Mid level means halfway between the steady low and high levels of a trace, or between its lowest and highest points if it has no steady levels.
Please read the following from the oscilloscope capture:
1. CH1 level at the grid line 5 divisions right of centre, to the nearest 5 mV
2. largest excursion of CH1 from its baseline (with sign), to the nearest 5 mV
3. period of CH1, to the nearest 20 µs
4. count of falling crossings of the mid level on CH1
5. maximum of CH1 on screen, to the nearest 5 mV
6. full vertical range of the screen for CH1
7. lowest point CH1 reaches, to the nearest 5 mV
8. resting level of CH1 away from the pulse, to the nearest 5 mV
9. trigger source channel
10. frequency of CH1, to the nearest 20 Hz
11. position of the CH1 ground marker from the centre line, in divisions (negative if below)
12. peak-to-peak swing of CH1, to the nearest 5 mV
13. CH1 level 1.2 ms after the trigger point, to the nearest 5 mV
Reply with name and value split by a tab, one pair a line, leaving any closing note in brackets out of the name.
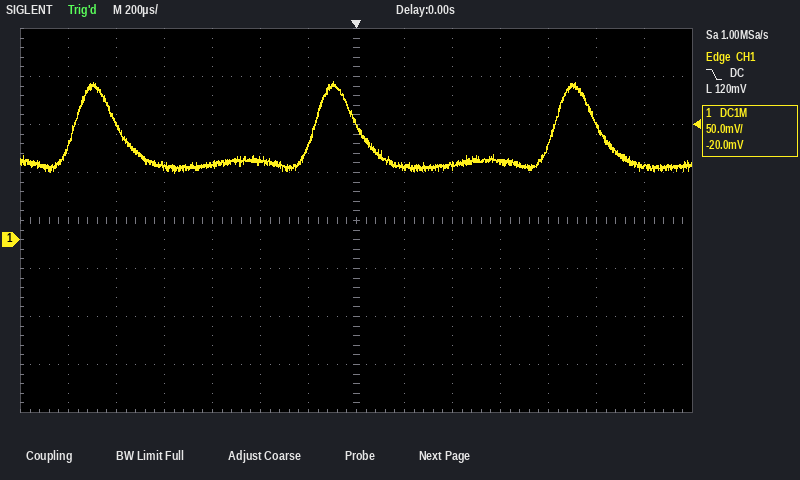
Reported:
CH1 level at the grid line 5 divisions right of centre, to the nearest 5 mV	120 mV
largest excursion of CH1 from its baseline (with sign), to the nearest 5 mV	+85 mV
period of CH1, to the nearest 20 µs	1.00 ms
count of falling crossings of the mid level on CH1	3
maximum of CH1 on screen, to the nearest 5 mV	165 mV
full vertical range of the screen for CH1	400 mV
lowest point CH1 reaches, to the nearest 5 mV	70 mV
resting level of CH1 away from the pulse, to the nearest 5 mV	80 mV
trigger source channel	CH1
frequency of CH1, to the nearest 20 Hz	1.00 kHz
position of the CH1 ground marker from the centre line, in divisions	-0.4 div
peak-to-peak swing of CH1, to the nearest 5 mV	95 mV
CH1 level 1.2 ms after the trigger point, to the nearest 5 mV	75 mV
